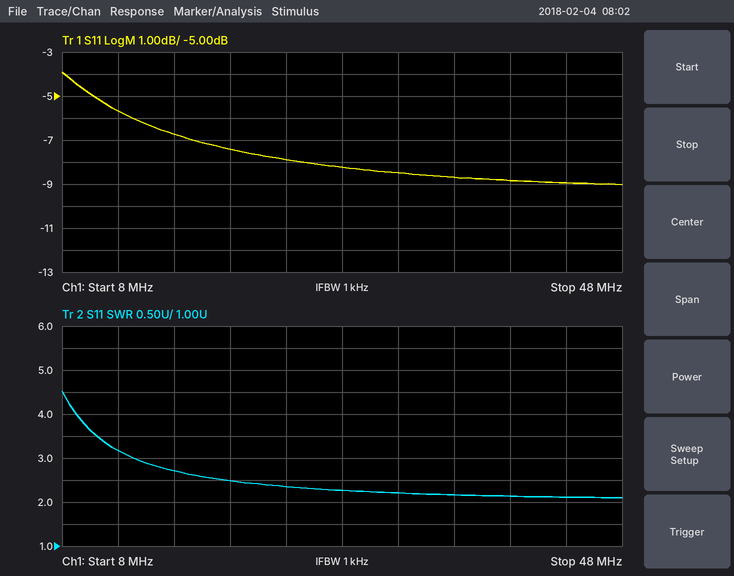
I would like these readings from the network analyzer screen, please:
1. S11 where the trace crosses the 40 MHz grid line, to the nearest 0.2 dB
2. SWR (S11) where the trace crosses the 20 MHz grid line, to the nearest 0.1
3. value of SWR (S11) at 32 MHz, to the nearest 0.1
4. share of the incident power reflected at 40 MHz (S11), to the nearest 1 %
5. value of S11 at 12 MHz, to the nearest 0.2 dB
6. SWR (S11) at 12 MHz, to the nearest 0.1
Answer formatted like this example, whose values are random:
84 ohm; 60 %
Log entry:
-8.8 dB; 2.5; 2.2; 13 %; -5.6 dB; 3.2
